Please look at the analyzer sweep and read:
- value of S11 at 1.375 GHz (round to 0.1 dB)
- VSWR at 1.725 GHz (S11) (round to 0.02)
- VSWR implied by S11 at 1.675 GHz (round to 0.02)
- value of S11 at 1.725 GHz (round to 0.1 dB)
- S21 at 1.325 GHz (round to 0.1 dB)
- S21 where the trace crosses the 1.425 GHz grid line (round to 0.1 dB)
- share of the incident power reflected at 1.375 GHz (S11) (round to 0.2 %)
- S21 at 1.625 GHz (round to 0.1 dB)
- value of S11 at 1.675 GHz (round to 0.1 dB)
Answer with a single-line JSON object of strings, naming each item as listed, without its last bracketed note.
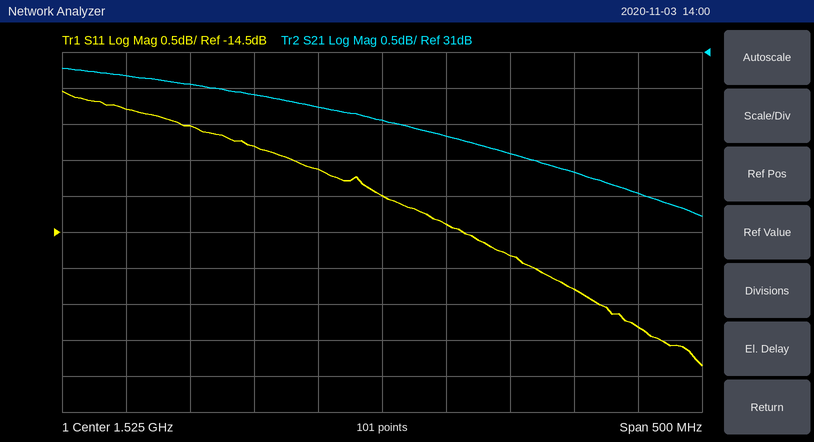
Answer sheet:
{"value of S11 at 1.375 GHz": "-13.0 dB", "VSWR at 1.725 GHz (S11)": "1.38", "VSWR implied by S11 at 1.675 GHz": "1.42", "value of S11 at 1.725 GHz": "-15.8 dB", "S21 at 1.325 GHz": "30.7 dB", "S21 where the trace crosses the 1.425 GHz grid line": "30.4 dB", "share of the incident power reflected at 1.375 GHz (S11)": "5.0 %", "S21 at 1.625 GHz": "29.6 dB", "value of S11 at 1.675 GHz": "-15.3 dB"}
